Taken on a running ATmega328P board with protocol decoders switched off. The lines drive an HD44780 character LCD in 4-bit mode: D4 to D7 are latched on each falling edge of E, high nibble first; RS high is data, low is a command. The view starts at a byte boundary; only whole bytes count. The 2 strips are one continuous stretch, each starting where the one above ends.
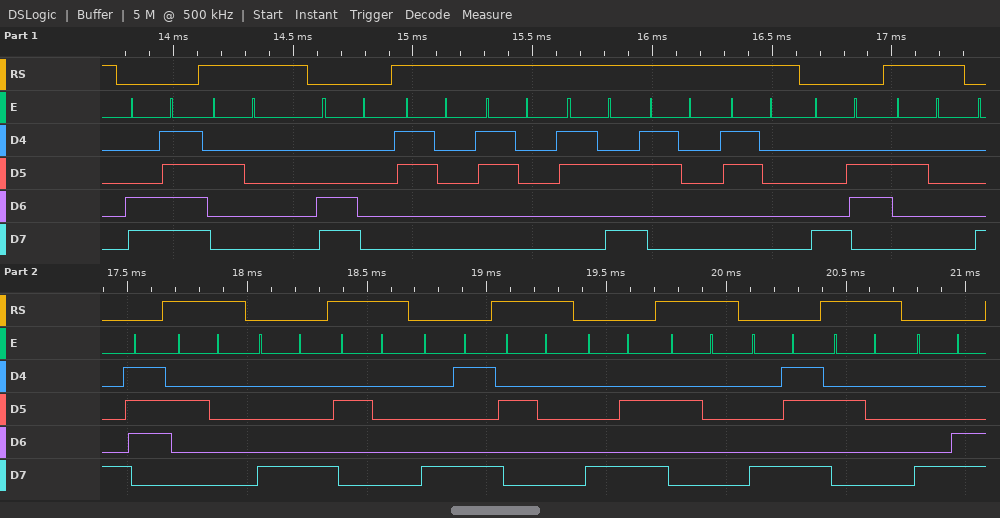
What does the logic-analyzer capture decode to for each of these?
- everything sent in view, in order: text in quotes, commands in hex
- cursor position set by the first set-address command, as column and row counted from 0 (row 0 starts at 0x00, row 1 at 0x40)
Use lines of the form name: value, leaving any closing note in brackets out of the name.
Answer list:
everything sent in view, in order: text in quotes, commands in hex: 0xCF " " 0xC0 "00:00" 0x86 " " 0x87 " " 0x88 " " 0x89 " " 0x8A " " 0x8B " " 0x8C
cursor position set by the first set-address command, as column and row counted from 0: column 15, row 1
